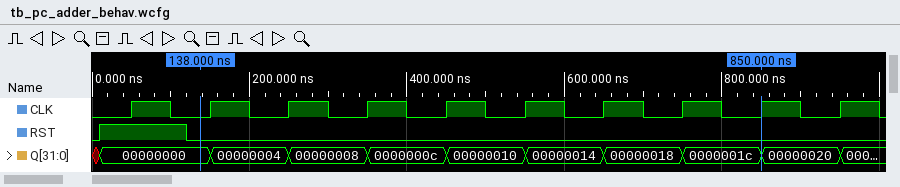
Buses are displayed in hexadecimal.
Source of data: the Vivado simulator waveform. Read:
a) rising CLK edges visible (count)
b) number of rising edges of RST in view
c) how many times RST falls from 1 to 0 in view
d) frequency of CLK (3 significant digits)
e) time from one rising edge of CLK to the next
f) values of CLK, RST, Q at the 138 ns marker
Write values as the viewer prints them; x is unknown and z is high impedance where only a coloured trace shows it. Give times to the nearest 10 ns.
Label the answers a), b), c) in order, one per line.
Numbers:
a) 10
b) 1
c) 1
d) 10.0 MHz
e) 100 ns
f) CLK=0, RST=0, Q=00000000
